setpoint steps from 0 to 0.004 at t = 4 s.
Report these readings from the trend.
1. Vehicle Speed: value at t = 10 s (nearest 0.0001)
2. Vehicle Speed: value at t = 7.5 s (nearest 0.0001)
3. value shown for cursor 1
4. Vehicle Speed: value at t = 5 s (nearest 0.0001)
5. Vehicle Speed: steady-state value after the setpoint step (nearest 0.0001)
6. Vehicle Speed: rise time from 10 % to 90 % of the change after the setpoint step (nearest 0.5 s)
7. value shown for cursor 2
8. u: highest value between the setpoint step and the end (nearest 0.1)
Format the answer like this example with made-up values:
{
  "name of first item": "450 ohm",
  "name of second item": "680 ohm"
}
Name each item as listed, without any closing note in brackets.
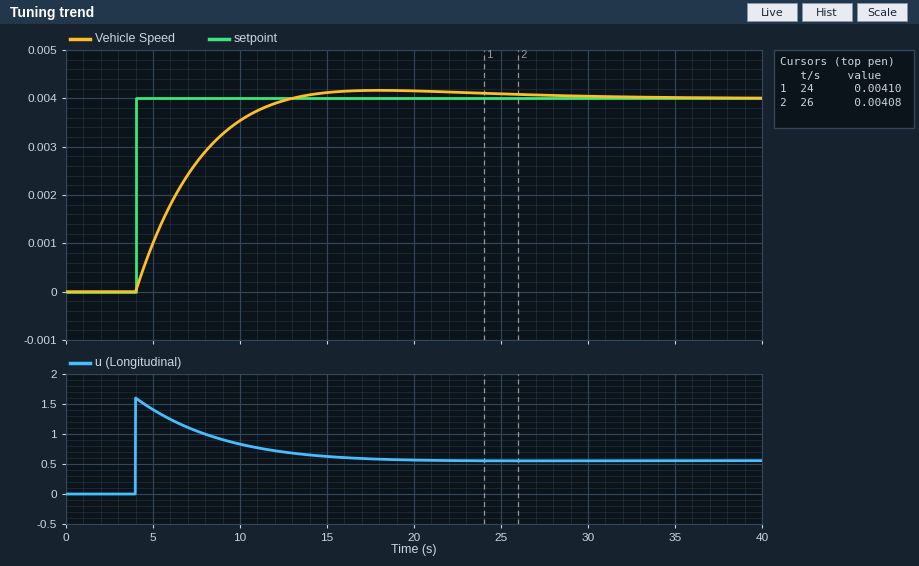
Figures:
{
  "Vehicle Speed: value at t = 10 s": "0.0035",
  "Vehicle Speed: value at t = 7.5 s": "0.0027",
  "value shown for cursor 1": "0.00410",
  "Vehicle Speed: value at t = 5 s": "0.0010",
  "Vehicle Speed: steady-state value after the setpoint step": "0.0040",
  "Vehicle Speed: rise time from 10 % to 90 % of the change after the setpoint step": "6.0 s",
  "value shown for cursor 2": "0.00408",
  "u: highest value between the setpoint step and the end": "1.6"
}
